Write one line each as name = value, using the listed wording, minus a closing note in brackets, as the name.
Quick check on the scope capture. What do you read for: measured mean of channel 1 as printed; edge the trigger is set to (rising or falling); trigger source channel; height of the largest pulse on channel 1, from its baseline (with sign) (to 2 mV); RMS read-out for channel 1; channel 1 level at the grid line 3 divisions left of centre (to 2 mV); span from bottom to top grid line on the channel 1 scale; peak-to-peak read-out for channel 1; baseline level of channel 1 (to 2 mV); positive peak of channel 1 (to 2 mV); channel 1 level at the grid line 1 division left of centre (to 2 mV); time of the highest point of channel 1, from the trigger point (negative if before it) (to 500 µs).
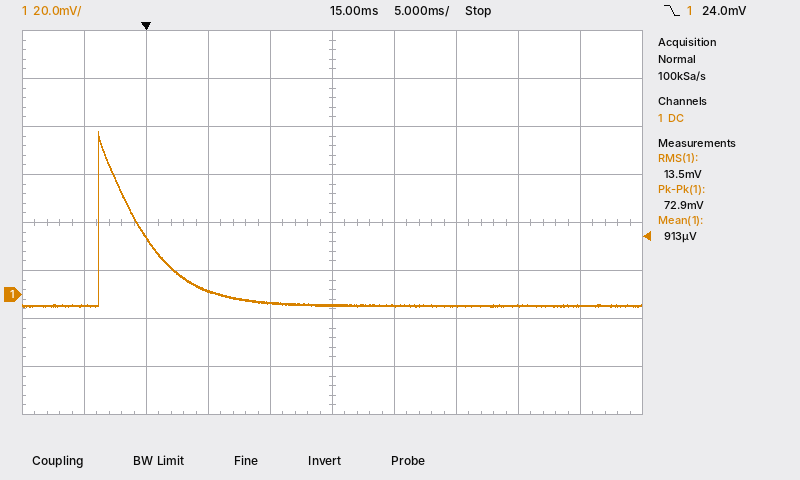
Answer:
measured mean of channel 1 as printed = 913 µV
edge the trigger is set to = falling
trigger source channel = channel 1
height of the largest pulse on channel 1, from its baseline (with sign) = +72 mV
RMS read-out for channel 1 = 13.5 mV
channel 1 level at the grid line 3 divisions left of centre = 24 mV
span from bottom to top grid line on the channel 1 scale = 160 mV
peak-to-peak read-out for channel 1 = 72.9 mV
baseline level of channel 1 = -4 mV
positive peak of channel 1 = 68 mV
channel 1 level at the grid line 1 division left of centre = -4 mV
time of the highest point of channel 1, from the trigger point (negative if before it) = -4.0 ms
